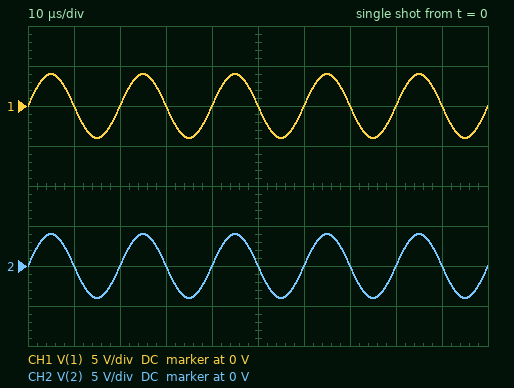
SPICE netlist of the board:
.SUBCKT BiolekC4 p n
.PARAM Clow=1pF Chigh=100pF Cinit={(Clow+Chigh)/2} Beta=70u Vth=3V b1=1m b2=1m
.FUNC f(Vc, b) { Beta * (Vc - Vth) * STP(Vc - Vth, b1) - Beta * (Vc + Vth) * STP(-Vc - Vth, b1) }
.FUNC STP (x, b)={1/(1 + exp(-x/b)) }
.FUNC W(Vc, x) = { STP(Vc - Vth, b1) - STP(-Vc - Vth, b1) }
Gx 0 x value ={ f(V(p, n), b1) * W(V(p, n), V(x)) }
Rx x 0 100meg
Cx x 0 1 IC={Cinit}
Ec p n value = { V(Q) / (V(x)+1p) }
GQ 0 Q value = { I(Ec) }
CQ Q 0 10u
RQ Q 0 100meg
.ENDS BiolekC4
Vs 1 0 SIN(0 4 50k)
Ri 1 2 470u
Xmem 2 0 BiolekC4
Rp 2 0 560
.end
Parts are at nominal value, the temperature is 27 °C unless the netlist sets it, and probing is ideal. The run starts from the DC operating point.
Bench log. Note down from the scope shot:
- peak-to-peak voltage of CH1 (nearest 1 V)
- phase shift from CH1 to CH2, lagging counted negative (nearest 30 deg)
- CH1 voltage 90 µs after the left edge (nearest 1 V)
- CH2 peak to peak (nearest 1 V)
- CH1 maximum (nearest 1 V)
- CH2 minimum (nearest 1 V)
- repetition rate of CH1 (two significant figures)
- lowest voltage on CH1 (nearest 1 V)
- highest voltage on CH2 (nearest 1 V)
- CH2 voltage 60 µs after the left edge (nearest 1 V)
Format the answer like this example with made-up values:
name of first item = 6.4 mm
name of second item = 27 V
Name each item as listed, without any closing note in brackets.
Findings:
peak-to-peak voltage of CH1 = 8 V
phase shift from CH1 to CH2, lagging counted negative = 0 deg
CH1 voltage 90 µs after the left edge = 0 V
CH2 peak to peak = 8 V
CH1 maximum = 4 V
CH2 minimum = -4 V
repetition rate of CH1 = 50 kHz
lowest voltage on CH1 = -4 V
highest voltage on CH2 = 4 V
CH2 voltage 60 µs after the left edge = 0 V
